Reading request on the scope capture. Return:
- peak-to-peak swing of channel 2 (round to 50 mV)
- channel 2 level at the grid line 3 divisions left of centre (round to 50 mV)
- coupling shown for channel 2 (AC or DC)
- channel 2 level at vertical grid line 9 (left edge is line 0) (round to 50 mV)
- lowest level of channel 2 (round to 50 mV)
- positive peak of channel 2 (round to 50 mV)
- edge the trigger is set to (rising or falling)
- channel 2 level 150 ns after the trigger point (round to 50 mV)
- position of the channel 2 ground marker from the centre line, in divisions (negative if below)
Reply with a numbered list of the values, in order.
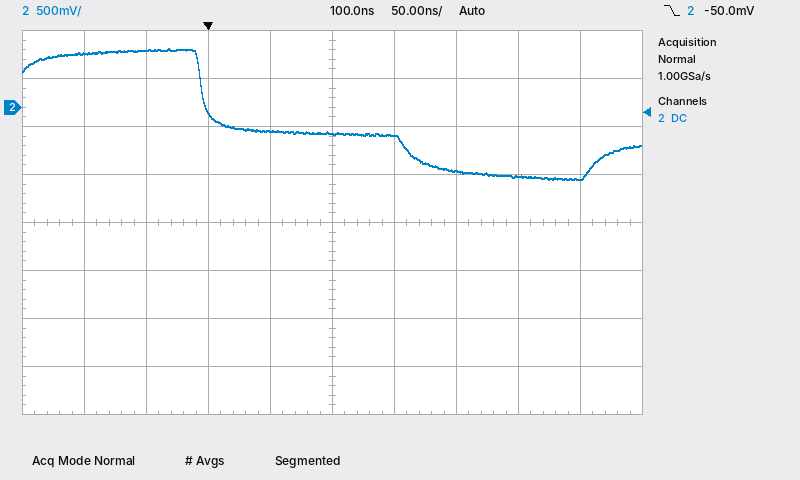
1. 1.35 V
2. 600 mV
3. DC
4. -750 mV
5. -750 mV
6. 600 mV
7. falling
8. -300 mV
9. +2.4 div
